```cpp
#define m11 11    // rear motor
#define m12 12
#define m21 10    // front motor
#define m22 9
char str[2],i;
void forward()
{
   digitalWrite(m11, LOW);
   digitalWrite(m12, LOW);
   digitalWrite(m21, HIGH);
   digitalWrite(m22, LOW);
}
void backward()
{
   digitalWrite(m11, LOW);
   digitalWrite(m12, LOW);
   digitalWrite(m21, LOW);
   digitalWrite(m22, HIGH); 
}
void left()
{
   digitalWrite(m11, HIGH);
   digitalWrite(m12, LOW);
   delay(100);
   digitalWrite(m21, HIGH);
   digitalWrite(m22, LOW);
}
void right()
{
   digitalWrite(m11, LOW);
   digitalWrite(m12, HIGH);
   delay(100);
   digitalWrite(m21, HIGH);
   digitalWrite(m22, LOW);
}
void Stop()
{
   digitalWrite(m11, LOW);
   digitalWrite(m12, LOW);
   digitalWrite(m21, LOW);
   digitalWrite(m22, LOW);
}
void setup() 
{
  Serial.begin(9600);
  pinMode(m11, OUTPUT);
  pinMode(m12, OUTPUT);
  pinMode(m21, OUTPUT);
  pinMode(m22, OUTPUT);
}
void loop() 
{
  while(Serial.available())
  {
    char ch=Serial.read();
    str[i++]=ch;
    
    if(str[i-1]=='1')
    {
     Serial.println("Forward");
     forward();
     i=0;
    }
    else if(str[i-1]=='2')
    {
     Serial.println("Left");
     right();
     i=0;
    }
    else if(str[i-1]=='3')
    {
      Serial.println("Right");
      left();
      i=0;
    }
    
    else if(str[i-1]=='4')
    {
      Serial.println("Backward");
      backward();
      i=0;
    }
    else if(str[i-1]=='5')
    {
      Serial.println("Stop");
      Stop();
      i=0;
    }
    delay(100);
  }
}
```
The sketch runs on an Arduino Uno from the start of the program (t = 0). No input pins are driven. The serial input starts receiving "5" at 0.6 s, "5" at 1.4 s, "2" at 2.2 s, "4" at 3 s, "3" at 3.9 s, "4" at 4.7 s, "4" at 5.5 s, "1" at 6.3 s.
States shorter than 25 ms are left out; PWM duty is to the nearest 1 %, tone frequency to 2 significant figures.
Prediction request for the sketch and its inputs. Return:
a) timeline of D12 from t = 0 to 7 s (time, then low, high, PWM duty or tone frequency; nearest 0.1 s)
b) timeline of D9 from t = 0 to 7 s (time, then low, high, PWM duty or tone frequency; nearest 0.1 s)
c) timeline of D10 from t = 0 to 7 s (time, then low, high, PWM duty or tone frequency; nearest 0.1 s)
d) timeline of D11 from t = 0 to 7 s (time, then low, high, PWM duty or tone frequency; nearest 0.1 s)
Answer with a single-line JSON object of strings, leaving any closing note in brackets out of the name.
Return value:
{"timeline of D12 from t = 0 to 7 s": "0 s low; 2.2 s high; 3 s low", "timeline of D9 from t = 0 to 7 s": "0 s low; 3 s high; 4 s low; 4.7 s high; 6.3 s low", "timeline of D10 from t = 0 to 7 s": "0 s low; 2.3 s high; 3 s low; 4 s high; 4.7 s low; 6.3 s high", "timeline of D11 from t = 0 to 7 s": "0 s low; 3.9 s high; 4.7 s low"}
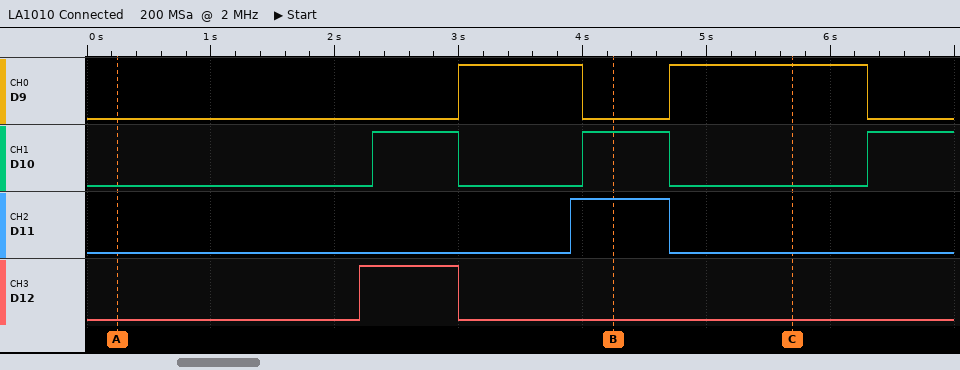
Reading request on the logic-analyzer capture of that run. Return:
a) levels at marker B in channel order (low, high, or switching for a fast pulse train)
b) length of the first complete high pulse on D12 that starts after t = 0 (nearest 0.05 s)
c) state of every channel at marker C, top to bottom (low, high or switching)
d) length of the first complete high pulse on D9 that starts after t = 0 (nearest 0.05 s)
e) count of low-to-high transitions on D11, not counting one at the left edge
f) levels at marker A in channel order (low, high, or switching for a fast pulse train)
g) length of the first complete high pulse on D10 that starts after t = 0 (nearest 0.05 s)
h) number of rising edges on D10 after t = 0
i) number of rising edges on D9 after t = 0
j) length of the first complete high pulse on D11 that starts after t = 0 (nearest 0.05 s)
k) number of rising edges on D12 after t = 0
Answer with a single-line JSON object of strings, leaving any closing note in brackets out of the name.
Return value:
{"levels at marker B in channel order": "D9 low, D10 high, D11 high, D12 low", "length of the first complete high pulse on D12 that starts after t = 0": "0.80 s", "state of every channel at marker C, top to bottom": "D9 high, D10 low, D11 low, D12 low", "length of the first complete high pulse on D9 that starts after t = 0": "1.00 s", "count of low-to-high transitions on D11, not counting one at the left edge": "1", "levels at marker A in channel order": "D9 low, D10 low, D11 low, D12 low", "length of the first complete high pulse on D10 that starts after t = 0": "0.70 s", "number of rising edges on D10 after t = 0": "3", "number of rising edges on D9 after t = 0": "2", "length of the first complete high pulse on D11 that starts after t = 0": "0.80 s", "number of rising edges on D12 after t = 0": "1"}
